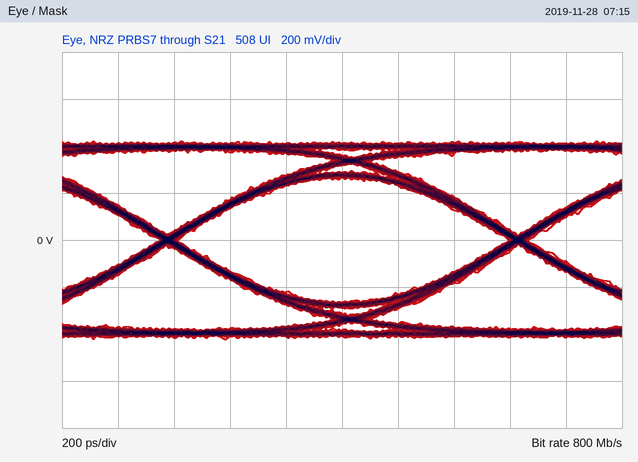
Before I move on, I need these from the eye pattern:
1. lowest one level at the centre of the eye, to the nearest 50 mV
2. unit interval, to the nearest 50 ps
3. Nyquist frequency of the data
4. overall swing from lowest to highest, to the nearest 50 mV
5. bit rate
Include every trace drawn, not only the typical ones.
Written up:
250 mV
1.25 ns
400 MHz
850 mV
800 Mb/s
